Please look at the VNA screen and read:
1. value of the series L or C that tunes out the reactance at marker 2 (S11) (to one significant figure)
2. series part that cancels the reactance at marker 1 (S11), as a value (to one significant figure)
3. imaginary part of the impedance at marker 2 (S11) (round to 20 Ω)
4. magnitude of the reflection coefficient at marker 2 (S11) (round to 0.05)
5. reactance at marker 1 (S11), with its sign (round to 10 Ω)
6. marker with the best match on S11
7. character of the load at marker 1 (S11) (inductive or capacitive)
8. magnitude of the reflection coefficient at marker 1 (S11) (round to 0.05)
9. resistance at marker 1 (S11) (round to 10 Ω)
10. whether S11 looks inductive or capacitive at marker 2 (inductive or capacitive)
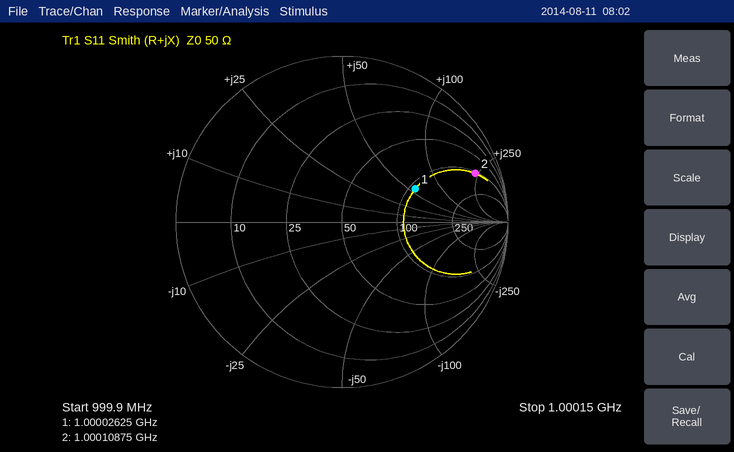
700 fF
3 pF
+240 Ω
0.85
+60 Ω
marker 1
inductive
0.50
110 Ω
inductive
